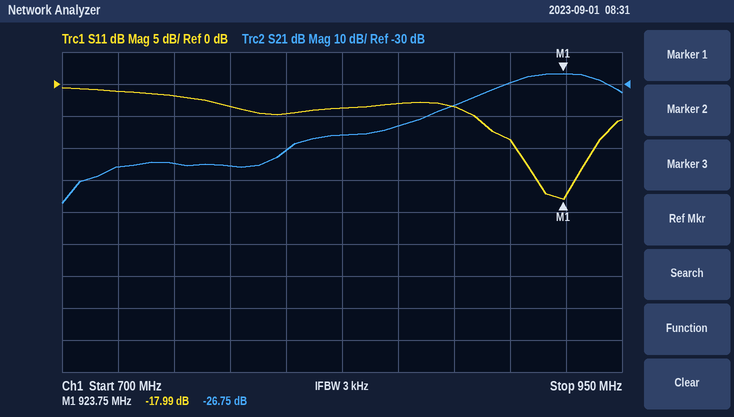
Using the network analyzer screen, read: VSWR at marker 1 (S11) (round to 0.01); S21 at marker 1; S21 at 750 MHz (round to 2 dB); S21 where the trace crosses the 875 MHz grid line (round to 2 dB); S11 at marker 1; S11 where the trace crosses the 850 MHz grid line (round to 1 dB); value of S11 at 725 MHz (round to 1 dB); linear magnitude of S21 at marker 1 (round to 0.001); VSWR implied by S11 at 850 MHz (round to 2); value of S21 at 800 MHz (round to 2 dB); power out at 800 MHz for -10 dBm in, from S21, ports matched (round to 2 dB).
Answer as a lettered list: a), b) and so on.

a) 1.29
b) -26.75 dB
c) -54 dB
d) -36 dB
e) -17.99 dB
f) -3 dB
g) -1 dB
h) 0.046
i) 6
j) -50 dB
k) -60 dBm
